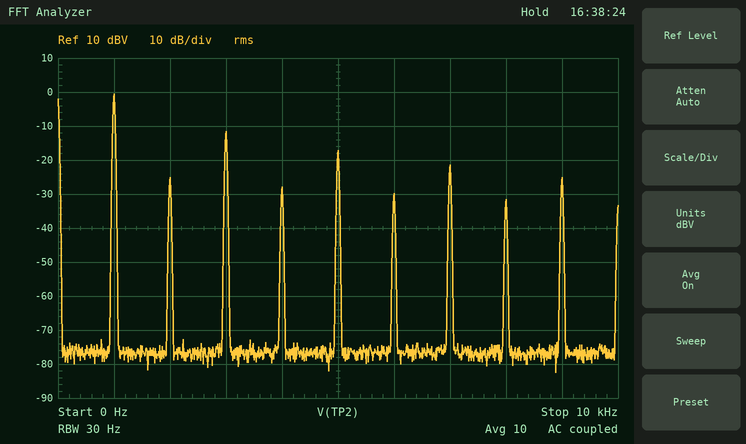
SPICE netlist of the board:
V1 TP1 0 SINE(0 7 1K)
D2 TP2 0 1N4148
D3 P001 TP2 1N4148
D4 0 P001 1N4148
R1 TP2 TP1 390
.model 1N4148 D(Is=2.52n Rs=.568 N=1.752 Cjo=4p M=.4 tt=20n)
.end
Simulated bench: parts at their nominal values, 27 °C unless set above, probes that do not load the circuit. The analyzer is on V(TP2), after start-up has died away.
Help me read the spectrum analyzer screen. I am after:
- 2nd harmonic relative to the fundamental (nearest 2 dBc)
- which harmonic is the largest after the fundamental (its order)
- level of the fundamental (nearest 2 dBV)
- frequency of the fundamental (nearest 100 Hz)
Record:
-24 dBc
3
0 dBV
1.0 kHz
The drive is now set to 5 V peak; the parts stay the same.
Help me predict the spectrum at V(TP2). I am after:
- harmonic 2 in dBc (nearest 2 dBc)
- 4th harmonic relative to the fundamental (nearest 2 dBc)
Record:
-22 dBc
-26 dBc
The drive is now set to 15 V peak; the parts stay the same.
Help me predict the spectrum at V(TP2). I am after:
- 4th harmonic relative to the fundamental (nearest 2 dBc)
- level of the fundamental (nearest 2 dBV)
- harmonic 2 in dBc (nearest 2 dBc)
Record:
-32 dBc
0 dBV
-28 dBc
